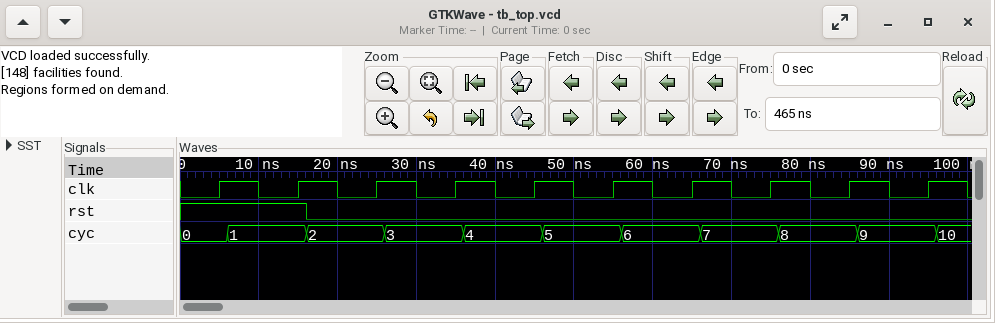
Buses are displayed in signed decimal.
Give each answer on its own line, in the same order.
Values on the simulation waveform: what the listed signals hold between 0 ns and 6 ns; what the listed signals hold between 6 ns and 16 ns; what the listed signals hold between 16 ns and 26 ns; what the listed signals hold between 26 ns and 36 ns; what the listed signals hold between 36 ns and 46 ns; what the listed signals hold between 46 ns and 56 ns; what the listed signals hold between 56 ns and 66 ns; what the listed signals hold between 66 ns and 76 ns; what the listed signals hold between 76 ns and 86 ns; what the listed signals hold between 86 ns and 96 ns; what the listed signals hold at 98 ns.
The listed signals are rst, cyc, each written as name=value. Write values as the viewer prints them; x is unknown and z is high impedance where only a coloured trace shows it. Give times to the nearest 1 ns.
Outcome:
rst=1, cyc=0
rst=1, cyc=1
rst=0, cyc=2
rst=0, cyc=3
rst=0, cyc=4
rst=0, cyc=5
rst=0, cyc=6
rst=0, cyc=7
rst=0, cyc=8
rst=0, cyc=9
rst=0, cyc=10
